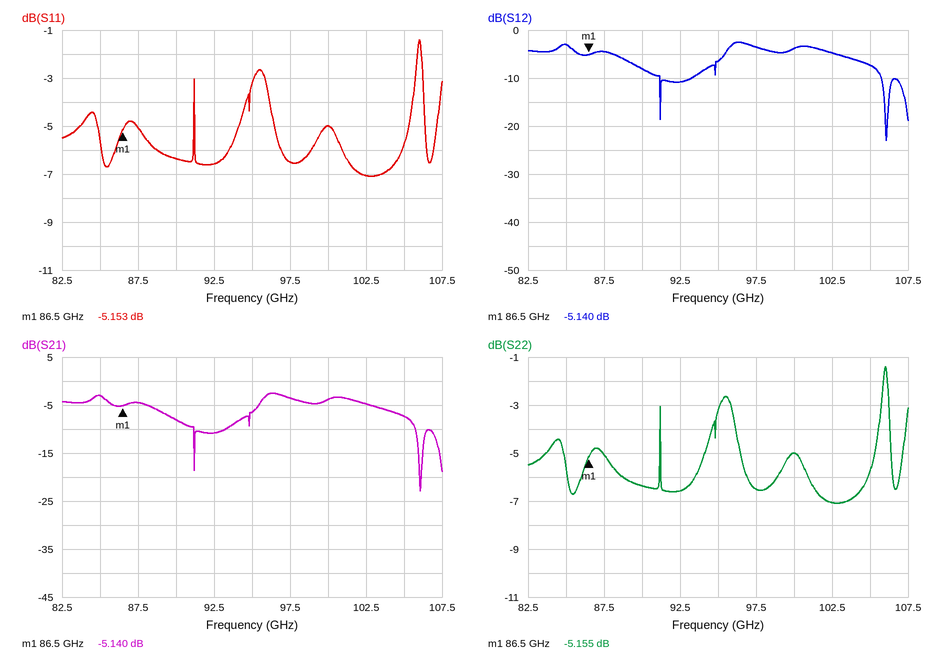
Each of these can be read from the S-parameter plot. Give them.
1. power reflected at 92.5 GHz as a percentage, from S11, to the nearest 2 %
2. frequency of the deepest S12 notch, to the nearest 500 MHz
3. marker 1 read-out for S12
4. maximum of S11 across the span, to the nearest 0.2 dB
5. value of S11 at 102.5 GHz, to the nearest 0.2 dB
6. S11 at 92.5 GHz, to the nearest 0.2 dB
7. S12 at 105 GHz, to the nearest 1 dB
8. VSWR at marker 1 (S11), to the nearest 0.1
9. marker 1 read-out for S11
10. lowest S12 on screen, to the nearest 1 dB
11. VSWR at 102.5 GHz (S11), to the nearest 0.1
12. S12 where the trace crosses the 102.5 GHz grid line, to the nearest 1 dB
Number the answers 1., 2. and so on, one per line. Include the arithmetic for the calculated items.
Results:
1. 10^(-6.6/10) ≈ 22 %
2. 106.0 GHz
3. -5.140 dB
4. -1.4 dB
5. -7.0 dB
6. -6.6 dB
7. -7 dB
8. (1 + 0.5525)/(1 − 0.5525) ≈ 3.5
9. -5.153 dB
10. -23 dB
11. |Γ| = 10^(-7/20) = 0.4467; VSWR = (1 + 0.4467)/(1 − 0.4467) ≈ 2.6
12. -5 dB
